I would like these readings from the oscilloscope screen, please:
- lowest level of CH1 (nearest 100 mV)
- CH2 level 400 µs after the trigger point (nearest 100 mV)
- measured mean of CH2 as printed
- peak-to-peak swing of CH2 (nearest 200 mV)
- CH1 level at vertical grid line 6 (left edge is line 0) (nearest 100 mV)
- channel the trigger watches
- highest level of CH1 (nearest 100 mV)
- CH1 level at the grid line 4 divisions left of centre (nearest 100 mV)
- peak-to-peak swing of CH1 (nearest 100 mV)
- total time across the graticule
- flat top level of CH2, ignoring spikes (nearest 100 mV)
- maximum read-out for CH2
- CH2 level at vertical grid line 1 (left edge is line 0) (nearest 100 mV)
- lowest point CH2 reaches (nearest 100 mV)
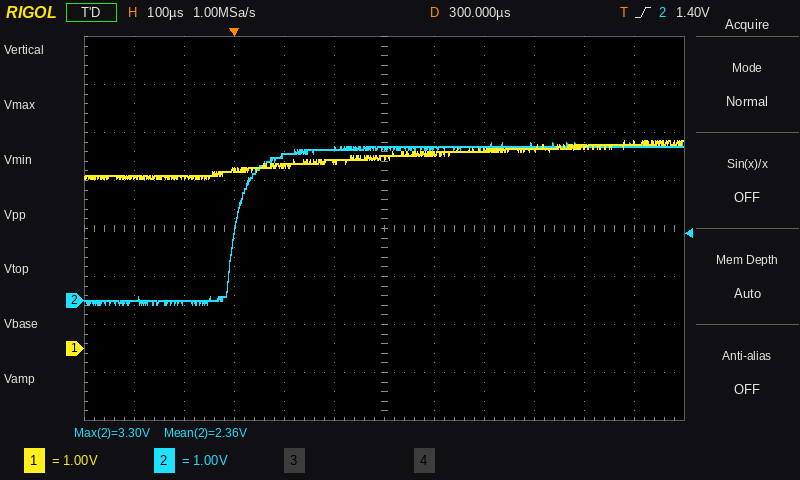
3.5 V
3.2 V
2.36 V
3.4 V
4.0 V
CH2
4.3 V
3.6 V
800 mV
1.2 ms
3.2 V
3.30 V
0.0 V
-100 mV
